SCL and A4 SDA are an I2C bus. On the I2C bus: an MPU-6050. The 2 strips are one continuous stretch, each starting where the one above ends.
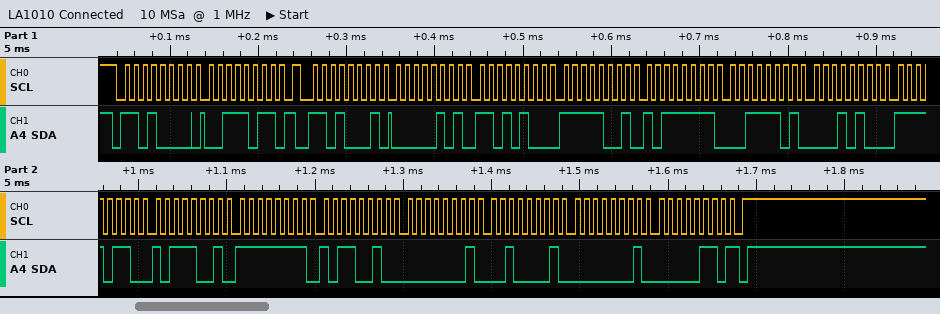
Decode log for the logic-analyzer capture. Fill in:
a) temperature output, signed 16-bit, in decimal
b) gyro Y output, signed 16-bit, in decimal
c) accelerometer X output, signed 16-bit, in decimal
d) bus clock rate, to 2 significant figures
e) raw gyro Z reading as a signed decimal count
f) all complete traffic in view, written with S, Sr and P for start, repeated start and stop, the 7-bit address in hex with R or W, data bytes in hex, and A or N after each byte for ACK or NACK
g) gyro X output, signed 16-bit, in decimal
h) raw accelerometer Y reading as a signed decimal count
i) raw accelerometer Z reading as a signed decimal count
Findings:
-2375
289
1492
100 kHz
262
S 68W A 3B A Sr 68R A 05 A D4 A F9 A BF A 3D A 14 A F6 A B9 A FF A B2 A 01 A 21 A 01 A 06 N P
-78
-1601
15636
